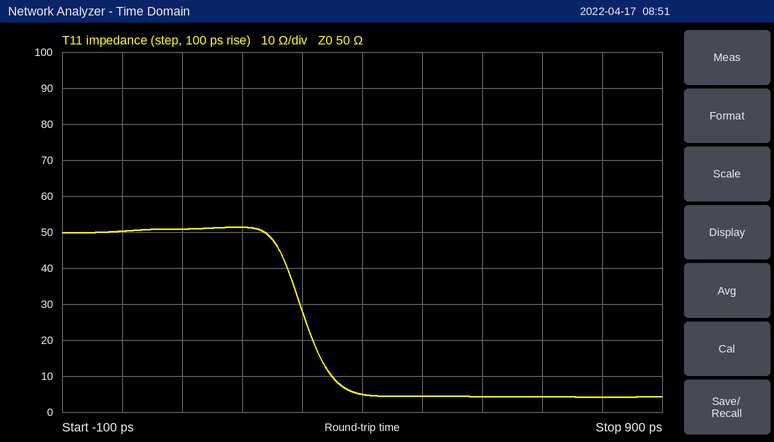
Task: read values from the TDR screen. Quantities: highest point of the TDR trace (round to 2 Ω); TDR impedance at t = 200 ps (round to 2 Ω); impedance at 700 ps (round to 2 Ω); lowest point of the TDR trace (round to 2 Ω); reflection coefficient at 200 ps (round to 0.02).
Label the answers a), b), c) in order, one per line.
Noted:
a) 52 Ω
b) 52 Ω
c) 4 Ω
d) 4 Ω
e) +0.02
